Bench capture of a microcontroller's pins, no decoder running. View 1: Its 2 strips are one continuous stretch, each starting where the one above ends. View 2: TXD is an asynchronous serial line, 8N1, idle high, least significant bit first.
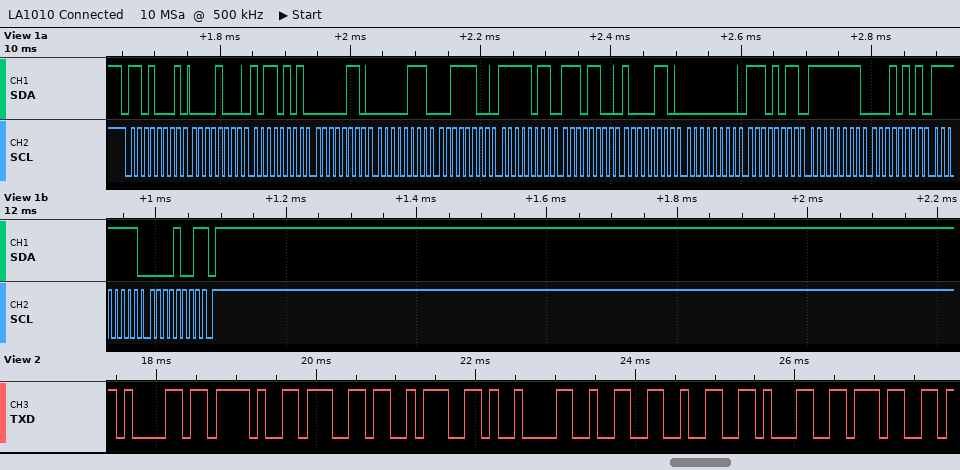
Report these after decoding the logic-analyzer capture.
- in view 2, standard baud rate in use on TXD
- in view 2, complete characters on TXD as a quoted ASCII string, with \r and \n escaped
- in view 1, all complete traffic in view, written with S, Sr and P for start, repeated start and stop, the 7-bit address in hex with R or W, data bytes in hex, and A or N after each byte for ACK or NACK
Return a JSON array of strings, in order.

["9600 baud", "\"a/g:\\t2217\"", "S 68R A 08 A B5 A 06 A 07 A 3C A FB A EC A 86 A 00 A EB A FF A 15 A FF A 09 N P"]
